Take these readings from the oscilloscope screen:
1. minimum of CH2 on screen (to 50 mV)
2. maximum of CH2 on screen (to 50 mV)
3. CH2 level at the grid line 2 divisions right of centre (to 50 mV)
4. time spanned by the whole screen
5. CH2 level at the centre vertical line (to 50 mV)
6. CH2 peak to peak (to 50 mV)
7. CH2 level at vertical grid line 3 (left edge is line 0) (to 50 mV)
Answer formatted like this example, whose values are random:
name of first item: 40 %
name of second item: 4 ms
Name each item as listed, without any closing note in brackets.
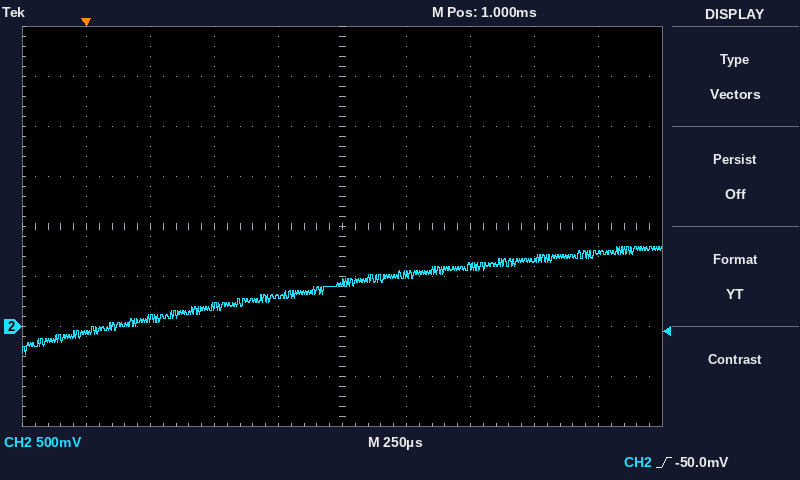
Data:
minimum of CH2 on screen: -300 mV
maximum of CH2 on screen: 800 mV
CH2 level at the grid line 2 divisions right of centre: 600 mV
time spanned by the whole screen: 2.5 ms
CH2 level at the centre vertical line: 450 mV
CH2 peak to peak: 1.10 V
CH2 level at vertical grid line 3 (left edge is line 0): 200 mV
